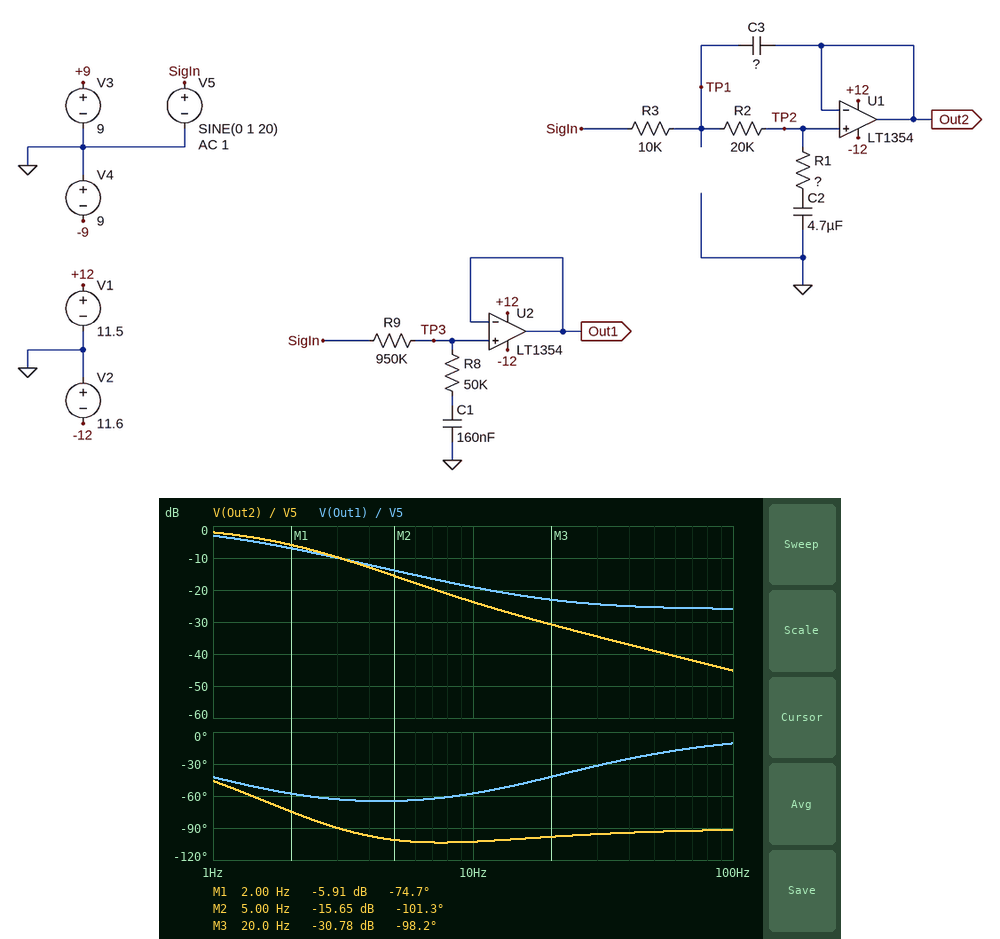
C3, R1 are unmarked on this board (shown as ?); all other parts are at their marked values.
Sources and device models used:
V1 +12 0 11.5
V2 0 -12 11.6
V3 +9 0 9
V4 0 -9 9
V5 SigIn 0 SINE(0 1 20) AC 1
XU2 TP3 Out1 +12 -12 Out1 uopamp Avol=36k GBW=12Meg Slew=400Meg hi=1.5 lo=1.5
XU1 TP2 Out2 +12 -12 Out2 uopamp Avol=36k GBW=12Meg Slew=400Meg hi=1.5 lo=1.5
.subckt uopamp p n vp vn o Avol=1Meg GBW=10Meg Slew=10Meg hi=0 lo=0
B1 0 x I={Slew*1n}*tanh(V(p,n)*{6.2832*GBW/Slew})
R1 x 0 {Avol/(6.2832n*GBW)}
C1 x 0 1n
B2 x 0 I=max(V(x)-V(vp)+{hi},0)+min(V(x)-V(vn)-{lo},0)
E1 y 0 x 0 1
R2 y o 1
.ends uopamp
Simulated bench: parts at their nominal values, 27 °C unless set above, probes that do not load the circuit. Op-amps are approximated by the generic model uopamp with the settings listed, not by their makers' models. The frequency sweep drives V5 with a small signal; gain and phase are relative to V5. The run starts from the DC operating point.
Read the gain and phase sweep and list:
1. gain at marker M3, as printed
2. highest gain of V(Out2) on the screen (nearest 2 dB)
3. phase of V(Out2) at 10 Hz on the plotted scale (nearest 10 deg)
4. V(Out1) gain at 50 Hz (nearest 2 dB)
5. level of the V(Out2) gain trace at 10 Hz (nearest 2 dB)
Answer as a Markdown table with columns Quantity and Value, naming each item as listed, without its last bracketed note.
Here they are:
| Quantity | Value |
|---|---|
| gain at marker M3, as printed | -30.78 dB |
| highest gain of V(Out2) on the screen | -2 dB |
| phase of V(Out2) at 10 Hz on the plotted scale | -100 deg |
| V(Out1) gain at 50 Hz | -26 dB |
| level of the V(Out2) gain trace at 10 Hz | -24 dB |
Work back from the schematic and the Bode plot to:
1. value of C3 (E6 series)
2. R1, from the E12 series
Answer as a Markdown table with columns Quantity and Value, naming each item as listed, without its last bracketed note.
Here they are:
| Quantity | Value |
|---|---|
| value of C3 | 6.8 µF |
| R1, from the E12 series | 4.7 kΩ |
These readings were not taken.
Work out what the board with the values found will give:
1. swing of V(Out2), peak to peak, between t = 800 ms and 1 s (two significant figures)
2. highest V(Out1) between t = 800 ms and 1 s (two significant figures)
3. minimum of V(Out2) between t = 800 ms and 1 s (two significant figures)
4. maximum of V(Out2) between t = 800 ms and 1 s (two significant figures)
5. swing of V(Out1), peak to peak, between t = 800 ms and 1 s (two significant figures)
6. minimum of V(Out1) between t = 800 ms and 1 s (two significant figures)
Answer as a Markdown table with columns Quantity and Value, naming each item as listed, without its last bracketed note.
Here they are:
| Quantity | Value |
|---|---|
| swing of V(Out2), peak to peak, between t = 800 ms and 1 s | 58 mV |
| highest V(Out1) between t = 800 ms and 1 s | 71 mV |
| minimum of V(Out2) between t = 800 ms and 1 s | -29 mV |
| maximum of V(Out2) between t = 800 ms and 1 s | 29 mV |
| swing of V(Out1), peak to peak, between t = 800 ms and 1 s | 140 mV |
| minimum of V(Out1) between t = 800 ms and 1 s | -70 mV |
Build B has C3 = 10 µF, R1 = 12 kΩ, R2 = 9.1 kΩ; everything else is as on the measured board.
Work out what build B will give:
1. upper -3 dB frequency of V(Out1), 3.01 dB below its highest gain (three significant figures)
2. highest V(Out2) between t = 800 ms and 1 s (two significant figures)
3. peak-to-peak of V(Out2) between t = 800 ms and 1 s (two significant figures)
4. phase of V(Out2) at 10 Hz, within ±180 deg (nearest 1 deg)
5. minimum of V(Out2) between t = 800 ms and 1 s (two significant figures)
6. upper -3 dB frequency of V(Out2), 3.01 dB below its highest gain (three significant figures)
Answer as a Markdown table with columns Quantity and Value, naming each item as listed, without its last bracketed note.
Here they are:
| Quantity | Value |
|---|---|
| upper -3 dB frequency of V(Out1), 3.01 dB below its highest gain | 997 mHz |
| highest V(Out2) between t = 800 ms and 1 s | 100 mV |
| peak-to-peak of V(Out2) between t = 800 ms and 1 s | 210 mV |
| phase of V(Out2) at 10 Hz, within ±180 deg | -76 deg |
| minimum of V(Out2) between t = 800 ms and 1 s | -100 mV |
| upper -3 dB frequency of V(Out2), 3.01 dB below its highest gain | 1.72 Hz |
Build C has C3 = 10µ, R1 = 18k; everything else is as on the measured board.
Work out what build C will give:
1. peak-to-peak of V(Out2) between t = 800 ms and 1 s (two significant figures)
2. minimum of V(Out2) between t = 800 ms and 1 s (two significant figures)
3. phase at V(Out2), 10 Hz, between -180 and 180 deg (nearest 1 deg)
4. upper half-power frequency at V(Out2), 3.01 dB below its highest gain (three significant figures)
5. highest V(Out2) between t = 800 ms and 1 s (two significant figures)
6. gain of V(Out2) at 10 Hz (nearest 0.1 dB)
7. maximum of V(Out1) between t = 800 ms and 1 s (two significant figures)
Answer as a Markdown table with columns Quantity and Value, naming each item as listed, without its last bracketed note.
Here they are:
| Quantity | Value |
|---|---|
| peak-to-peak of V(Out2) between t = 800 ms and 1 s | 140 mV |
| minimum of V(Out2) between t = 800 ms and 1 s | -71 mV |
| phase at V(Out2), 10 Hz, between -180 and 180 deg | -79 deg |
| upper half-power frequency at V(Out2), 3.01 dB below its highest gain | 1.08 Hz |
| highest V(Out2) between t = 800 ms and 1 s | 71 mV |
| gain of V(Out2) at 10 Hz | -17.1 dB |
| maximum of V(Out1) between t = 800 ms and 1 s | 71 mV |
